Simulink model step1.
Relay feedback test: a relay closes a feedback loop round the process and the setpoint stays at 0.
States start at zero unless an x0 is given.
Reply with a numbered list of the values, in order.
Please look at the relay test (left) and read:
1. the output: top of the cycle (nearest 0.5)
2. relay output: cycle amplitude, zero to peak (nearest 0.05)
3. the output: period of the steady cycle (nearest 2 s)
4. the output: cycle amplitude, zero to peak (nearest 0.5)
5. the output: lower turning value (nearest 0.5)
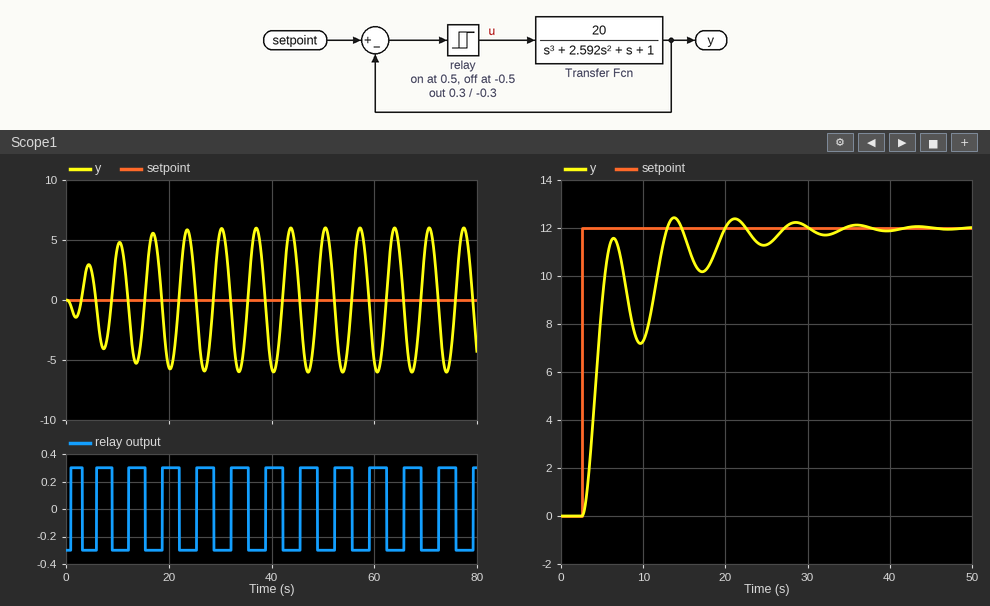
1. 6.0
2. 0.30
3. 6 s
4. 6.0
5. -6.0
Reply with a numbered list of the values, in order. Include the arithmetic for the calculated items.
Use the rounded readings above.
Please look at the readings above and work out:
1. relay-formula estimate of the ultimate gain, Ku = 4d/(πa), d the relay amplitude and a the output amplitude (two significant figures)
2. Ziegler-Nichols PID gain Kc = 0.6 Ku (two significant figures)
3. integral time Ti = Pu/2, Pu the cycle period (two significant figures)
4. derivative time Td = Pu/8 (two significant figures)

1. 4 × 0.3 / (π × 6) = 0.064
2. 0.6 × 0.064 = 0.038
3. 6 / 2 = 3.0 s
4. 6 / 8 = 0.75 s
